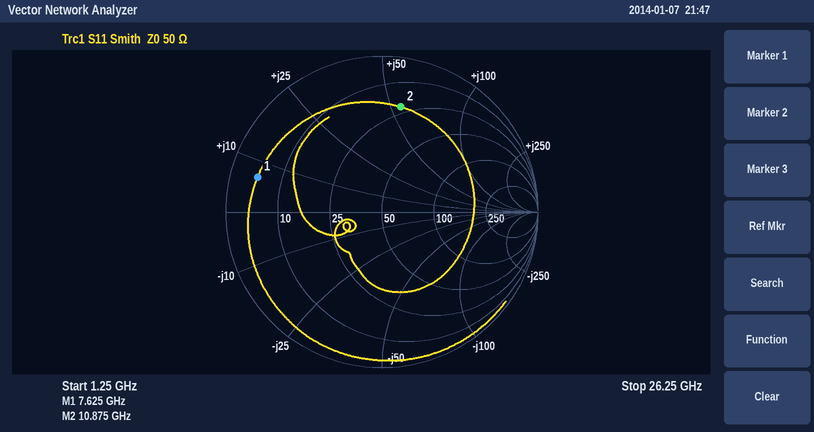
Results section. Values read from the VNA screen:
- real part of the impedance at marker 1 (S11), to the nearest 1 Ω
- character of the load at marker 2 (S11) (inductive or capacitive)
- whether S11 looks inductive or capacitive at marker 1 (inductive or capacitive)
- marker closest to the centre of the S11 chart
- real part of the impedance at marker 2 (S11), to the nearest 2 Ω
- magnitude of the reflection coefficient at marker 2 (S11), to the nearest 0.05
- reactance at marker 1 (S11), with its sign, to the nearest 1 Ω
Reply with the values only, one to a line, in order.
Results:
5 Ω
inductive
inductive
marker 2
22 Ω
0.70
+7 Ω
